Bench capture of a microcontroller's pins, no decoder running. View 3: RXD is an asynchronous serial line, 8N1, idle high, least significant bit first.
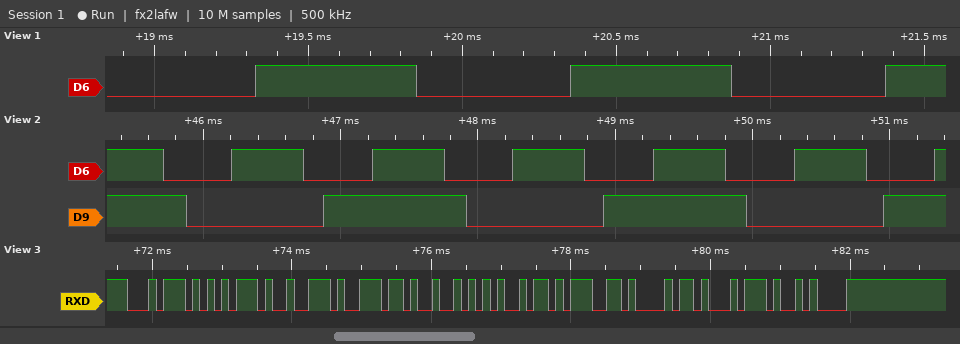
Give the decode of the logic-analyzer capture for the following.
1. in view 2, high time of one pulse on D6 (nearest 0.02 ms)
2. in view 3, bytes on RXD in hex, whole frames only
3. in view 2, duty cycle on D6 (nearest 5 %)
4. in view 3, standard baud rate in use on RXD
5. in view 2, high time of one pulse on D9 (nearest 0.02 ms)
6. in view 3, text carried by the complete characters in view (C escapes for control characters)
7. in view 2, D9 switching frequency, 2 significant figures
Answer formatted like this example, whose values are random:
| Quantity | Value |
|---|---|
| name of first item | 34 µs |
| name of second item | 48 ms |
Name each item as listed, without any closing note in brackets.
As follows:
| Quantity | Value |
|---|---|
| in view 2, high time of one pulse on D6 | 0.52 ms |
| in view 3, bytes on RXD in hex, whole frames only | 0x74 0x75 0x72 0x6E 0x52 0x69 0x67 0x68 0x74 0x0A |
| in view 2, duty cycle on D6 | 50 % |
| in view 3, standard baud rate in use on RXD | 9600 baud |
| in view 2, high time of one pulse on D9 | 1.04 ms |
| in view 3, text carried by the complete characters in view | "turnRight\n" |
| in view 2, D9 switching frequency, 2 significant figures | 490 Hz |
